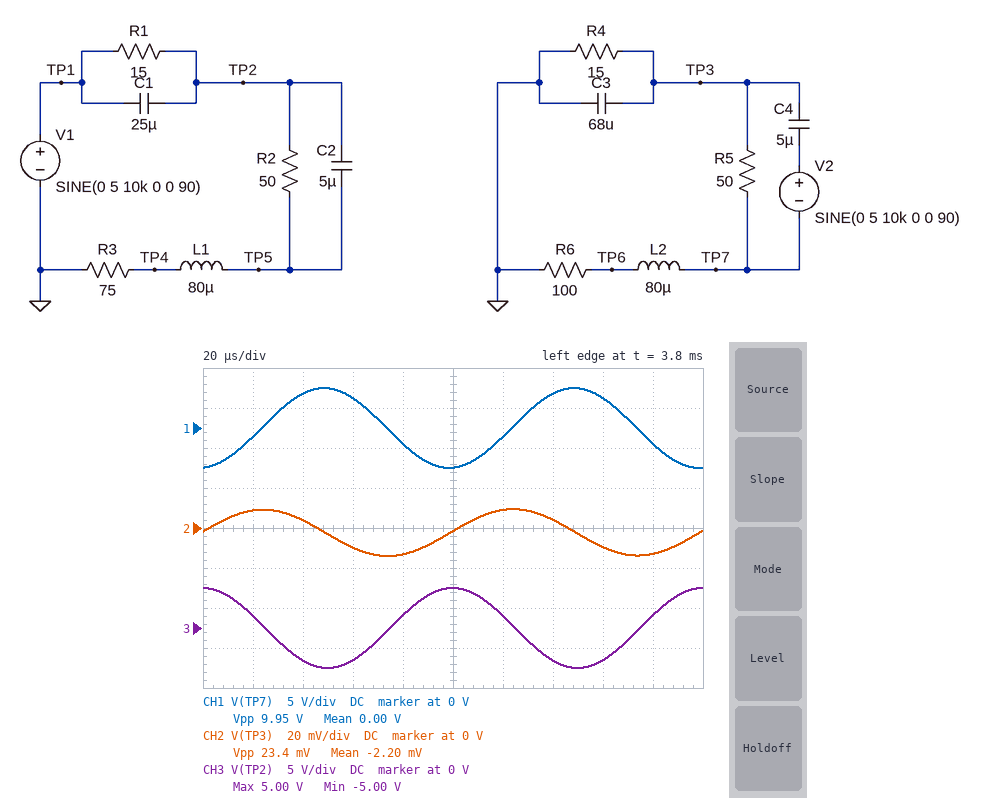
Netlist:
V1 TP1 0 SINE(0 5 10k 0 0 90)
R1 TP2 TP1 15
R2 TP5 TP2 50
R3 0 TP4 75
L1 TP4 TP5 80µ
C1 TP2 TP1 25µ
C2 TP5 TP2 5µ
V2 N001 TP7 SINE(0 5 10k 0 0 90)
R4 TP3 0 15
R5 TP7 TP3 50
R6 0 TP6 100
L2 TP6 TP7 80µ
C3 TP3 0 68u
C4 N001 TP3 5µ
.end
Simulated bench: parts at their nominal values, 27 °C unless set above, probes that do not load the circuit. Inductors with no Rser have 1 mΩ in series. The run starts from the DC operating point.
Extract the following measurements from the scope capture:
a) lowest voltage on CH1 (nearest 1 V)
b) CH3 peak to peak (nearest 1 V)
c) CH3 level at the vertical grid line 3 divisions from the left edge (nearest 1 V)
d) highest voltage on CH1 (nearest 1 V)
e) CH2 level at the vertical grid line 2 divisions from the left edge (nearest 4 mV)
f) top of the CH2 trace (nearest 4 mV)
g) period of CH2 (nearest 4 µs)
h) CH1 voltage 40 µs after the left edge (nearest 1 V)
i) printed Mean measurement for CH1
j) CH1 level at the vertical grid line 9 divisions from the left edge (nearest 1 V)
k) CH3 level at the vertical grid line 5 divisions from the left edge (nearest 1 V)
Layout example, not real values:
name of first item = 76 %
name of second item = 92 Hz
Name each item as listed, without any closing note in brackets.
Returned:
lowest voltage on CH1 = -5 V
CH3 peak to peak = 10 V
CH3 level at the vertical grid line 3 divisions from the left edge = -4 V
highest voltage on CH1 = 5 V
CH2 level at the vertical grid line 2 divisions from the left edge = 4 mV
top of the CH2 trace = 8 mV
period of CH2 = 100 µs
CH1 voltage 40 µs after the left edge = 4 V
printed Mean measurement for CH1 = 0.00 V
CH1 level at the vertical grid line 9 divisions from the left edge = -2 V
CH3 level at the vertical grid line 5 divisions from the left edge = 5 V
